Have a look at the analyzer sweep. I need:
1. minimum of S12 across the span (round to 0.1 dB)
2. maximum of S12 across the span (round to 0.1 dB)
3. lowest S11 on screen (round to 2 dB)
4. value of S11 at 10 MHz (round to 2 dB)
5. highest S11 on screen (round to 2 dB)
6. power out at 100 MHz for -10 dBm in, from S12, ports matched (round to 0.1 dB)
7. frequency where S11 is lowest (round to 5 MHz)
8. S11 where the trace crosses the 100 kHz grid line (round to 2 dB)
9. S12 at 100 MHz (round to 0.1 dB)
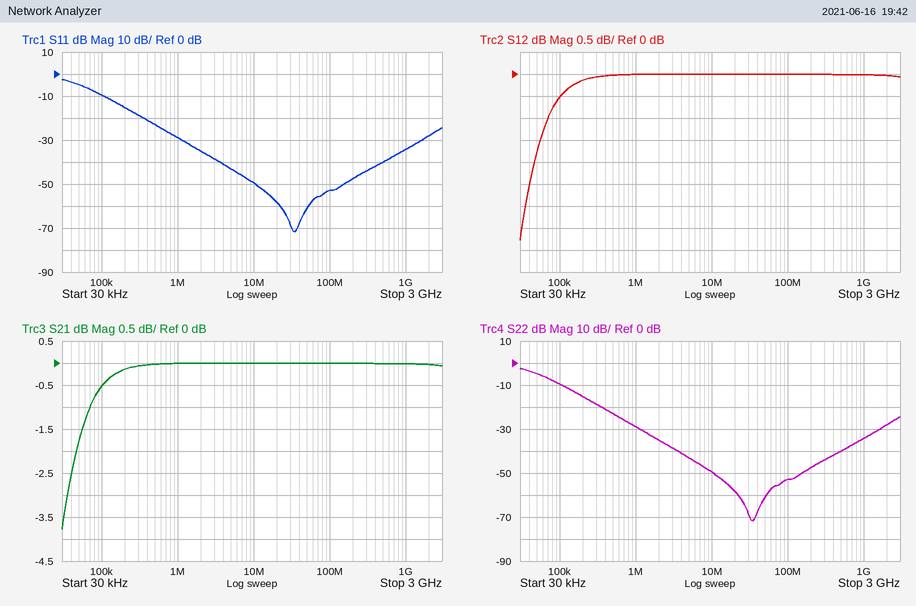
-3.8 dB
0.0 dB
-72 dB
-50 dB
-2 dB
-10.0 dBm
35 MHz
-10 dB
0.0 dB
